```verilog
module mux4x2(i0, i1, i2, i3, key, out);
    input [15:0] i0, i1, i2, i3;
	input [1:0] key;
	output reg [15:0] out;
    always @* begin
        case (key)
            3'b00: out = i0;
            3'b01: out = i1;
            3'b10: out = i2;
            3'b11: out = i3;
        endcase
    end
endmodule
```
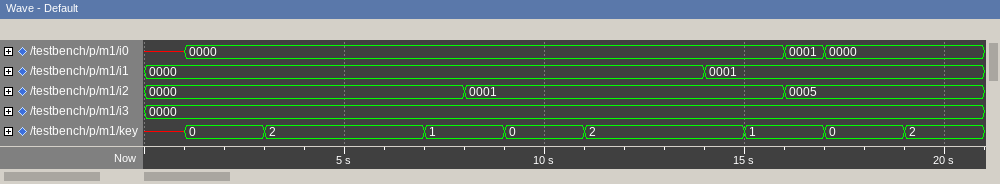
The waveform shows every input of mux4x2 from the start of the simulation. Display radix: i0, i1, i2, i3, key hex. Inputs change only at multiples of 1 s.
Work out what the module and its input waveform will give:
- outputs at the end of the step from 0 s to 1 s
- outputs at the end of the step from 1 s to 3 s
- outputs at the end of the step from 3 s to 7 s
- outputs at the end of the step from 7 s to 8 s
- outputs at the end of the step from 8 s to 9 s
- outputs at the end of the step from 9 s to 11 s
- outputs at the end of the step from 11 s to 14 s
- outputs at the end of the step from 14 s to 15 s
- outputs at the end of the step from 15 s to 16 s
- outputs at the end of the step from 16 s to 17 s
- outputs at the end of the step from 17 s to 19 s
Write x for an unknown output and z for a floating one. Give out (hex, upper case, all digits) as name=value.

out=x
out=0000
out=0000
out=0000
out=0000
out=0000
out=0001
out=0001
out=0001
out=0001
out=0000
